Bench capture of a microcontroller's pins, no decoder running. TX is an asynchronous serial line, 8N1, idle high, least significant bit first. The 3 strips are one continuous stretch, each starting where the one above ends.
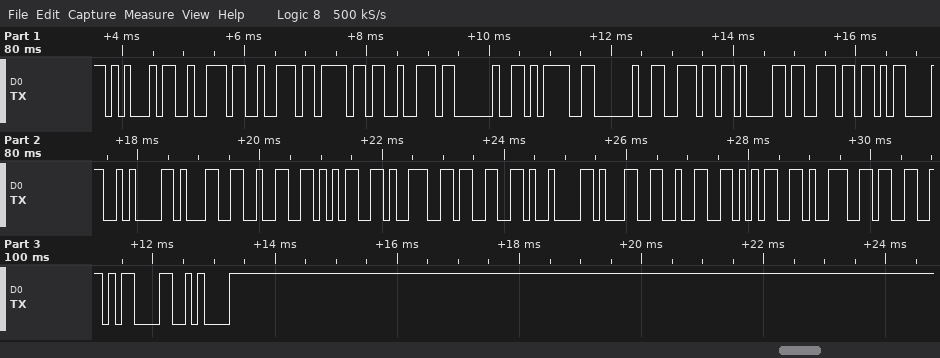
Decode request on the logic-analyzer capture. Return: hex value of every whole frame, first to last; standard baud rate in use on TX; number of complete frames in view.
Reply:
0x45 0x72 0x72 0x6F 0x72 0x20 0x3D 0x20 0x6E 0x61 0x6E 0x0D 0x0A 0x31 0x32 0x35 0x39 0x33 0x09 0x31 0x32 0x35 0x39 0x33 0x0D 0x0A
9600 baud
26
